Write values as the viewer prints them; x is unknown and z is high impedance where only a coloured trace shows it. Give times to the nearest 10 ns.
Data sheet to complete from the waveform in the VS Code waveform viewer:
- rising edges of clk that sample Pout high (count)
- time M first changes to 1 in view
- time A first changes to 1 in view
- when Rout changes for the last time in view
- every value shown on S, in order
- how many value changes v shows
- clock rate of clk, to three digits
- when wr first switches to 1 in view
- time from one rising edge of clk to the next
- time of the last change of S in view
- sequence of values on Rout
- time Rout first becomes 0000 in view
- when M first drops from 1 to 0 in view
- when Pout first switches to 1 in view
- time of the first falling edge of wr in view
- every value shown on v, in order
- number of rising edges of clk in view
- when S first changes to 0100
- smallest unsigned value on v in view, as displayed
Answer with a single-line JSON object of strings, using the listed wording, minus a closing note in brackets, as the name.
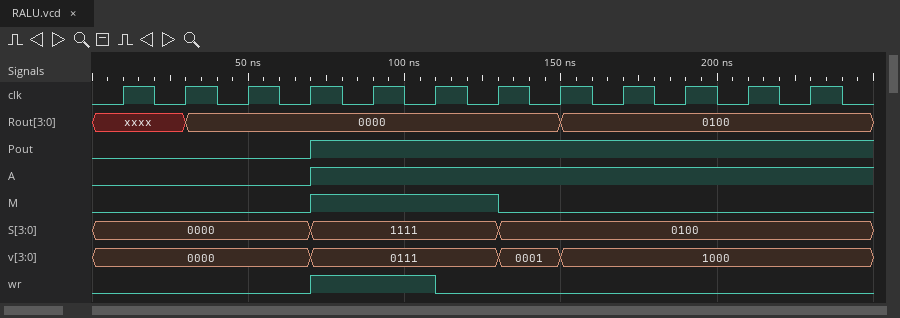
{"rising edges of clk that sample Pout high": "8", "time M first changes to 1 in view": "70 ns", "time A first changes to 1 in view": "70 ns", "when Rout changes for the last time in view": "150 ns", "every value shown on S, in order": "0000, 1111, 0100", "how many value changes v shows": "3", "clock rate of clk, to three digits": "50.0 MHz", "when wr first switches to 1 in view": "70 ns", "time from one rising edge of clk to the next": "20 ns", "time of the last change of S in view": "130 ns", "sequence of values on Rout": "xxxx, 0000, 0100", "time Rout first becomes 0000 in view": "30 ns", "when M first drops from 1 to 0 in view": "130 ns", "when Pout first switches to 1 in view": "70 ns", "time of the first falling edge of wr in view": "110 ns", "every value shown on v, in order": "0000, 0111, 0001, 1000", "number of rising edges of clk in view": "12", "when S first changes to 0100": "130 ns", "smallest unsigned value on v in view, as displayed": "0000"}
